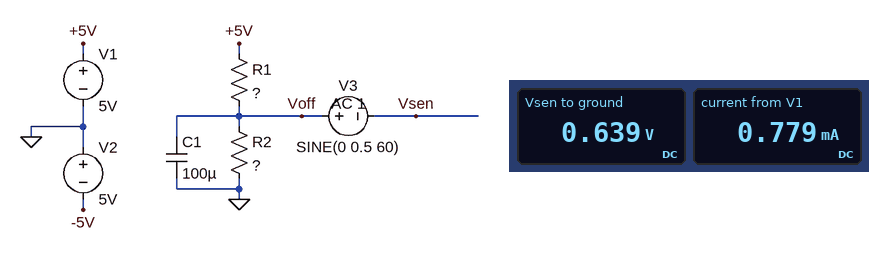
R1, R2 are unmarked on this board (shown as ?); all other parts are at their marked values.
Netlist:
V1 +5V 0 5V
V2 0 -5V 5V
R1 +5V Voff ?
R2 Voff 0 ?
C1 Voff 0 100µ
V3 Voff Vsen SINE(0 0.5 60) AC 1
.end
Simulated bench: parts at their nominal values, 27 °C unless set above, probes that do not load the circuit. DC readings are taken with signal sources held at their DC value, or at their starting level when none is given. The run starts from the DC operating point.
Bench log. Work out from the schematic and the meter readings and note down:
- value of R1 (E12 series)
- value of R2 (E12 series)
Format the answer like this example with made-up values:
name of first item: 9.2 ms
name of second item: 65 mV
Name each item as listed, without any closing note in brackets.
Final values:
value of R1: 5.6 kΩ
value of R2: 820 Ω
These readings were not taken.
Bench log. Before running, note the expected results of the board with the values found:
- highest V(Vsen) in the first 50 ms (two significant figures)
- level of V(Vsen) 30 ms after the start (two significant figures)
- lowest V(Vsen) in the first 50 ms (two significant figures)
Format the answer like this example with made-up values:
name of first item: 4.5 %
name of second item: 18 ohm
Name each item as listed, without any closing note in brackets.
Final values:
highest V(Vsen) in the first 50 ms: 1.1 V
level of V(Vsen) 30 ms after the start: 1.1 V
lowest V(Vsen) in the first 50 ms: 140 mV
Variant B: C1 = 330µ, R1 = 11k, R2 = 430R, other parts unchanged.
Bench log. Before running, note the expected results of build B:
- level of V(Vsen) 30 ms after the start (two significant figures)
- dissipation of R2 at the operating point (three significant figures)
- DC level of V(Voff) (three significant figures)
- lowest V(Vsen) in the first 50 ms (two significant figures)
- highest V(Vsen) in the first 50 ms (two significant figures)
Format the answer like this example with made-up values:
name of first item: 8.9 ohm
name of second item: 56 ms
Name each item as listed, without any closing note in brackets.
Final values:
level of V(Vsen) 30 ms after the start: 660 mV
dissipation of R2 at the operating point: 82.3 µW
DC level of V(Voff): 188 mV
lowest V(Vsen) in the first 50 ms: -310 mV
highest V(Vsen) in the first 50 ms: 690 mV
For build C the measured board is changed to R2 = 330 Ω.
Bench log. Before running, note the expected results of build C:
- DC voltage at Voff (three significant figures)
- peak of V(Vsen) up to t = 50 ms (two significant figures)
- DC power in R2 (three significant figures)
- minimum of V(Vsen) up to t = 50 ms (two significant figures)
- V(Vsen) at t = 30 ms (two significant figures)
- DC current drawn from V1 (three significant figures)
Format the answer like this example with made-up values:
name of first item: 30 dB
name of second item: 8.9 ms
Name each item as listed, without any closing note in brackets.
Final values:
DC voltage at Voff: 278 mV
peak of V(Vsen) up to t = 50 ms: 780 mV
DC power in R2: 235 µW
minimum of V(Vsen) up to t = 50 ms: -220 mV
V(Vsen) at t = 30 ms: 750 mV
DC current drawn from V1: 843 µA
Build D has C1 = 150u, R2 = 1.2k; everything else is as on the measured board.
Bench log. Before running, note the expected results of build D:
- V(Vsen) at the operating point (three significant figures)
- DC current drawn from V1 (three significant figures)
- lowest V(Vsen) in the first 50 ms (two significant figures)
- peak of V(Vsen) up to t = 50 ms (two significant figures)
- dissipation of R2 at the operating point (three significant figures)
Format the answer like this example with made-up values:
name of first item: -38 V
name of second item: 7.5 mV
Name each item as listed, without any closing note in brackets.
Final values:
V(Vsen) at the operating point: 882 mV
DC current drawn from V1: 735 µA
lowest V(Vsen) in the first 50 ms: 380 mV
peak of V(Vsen) up to t = 50 ms: 1.4 V
dissipation of R2 at the operating point: 649 µW
